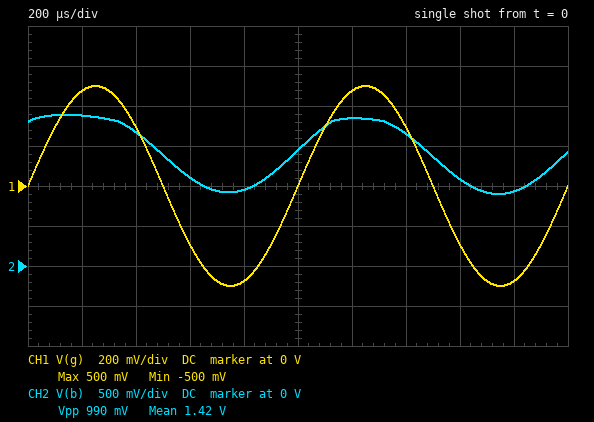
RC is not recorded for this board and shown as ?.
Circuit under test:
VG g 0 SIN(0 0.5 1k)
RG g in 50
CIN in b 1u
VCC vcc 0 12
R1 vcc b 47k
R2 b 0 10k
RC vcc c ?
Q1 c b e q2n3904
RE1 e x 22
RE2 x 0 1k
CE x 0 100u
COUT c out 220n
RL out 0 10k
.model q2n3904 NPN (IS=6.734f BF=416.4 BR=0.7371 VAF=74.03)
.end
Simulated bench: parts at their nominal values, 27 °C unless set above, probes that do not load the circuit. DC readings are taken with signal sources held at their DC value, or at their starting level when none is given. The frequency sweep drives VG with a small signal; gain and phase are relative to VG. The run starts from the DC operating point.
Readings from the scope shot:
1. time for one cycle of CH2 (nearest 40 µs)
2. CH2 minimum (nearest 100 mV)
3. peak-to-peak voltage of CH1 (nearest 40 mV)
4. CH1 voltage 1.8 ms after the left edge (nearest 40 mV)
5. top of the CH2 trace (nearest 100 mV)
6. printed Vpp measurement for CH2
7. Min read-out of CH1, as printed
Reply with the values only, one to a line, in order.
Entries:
1.00 ms
900 mV
1.00 V
-480 mV
1.9 V
990 mV
-500 mV
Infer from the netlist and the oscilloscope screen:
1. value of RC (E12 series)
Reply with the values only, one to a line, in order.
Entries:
10 kΩ
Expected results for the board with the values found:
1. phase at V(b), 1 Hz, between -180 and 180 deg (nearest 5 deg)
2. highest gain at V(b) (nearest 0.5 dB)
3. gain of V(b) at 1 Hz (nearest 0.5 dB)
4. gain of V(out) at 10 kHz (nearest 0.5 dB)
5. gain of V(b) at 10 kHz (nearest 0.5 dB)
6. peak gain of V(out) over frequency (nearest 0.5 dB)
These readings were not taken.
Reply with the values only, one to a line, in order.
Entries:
65 deg
-5.0 dB
-46.0 dB
15.5 dB
-5.0 dB
15.5 dB
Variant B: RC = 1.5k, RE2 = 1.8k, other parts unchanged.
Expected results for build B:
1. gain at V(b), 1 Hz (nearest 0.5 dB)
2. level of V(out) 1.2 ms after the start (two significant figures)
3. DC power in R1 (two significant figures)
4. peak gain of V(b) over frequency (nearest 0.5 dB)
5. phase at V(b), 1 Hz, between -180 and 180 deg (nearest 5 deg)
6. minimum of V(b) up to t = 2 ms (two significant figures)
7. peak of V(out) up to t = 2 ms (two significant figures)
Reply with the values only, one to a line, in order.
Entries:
-26.0 dB
-8.1 V
2.1 mW
0 dB
85 deg
1.4 V
2.3 V
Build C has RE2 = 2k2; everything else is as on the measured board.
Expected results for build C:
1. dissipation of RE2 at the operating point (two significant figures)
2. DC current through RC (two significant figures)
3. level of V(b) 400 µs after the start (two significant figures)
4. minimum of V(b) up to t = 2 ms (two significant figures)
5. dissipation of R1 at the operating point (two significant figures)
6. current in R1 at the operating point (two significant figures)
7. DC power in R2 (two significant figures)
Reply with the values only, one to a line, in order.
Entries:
920 µW
650 µA
2.0 V
1.2 V
2.1 mW
210 µA
440 µW
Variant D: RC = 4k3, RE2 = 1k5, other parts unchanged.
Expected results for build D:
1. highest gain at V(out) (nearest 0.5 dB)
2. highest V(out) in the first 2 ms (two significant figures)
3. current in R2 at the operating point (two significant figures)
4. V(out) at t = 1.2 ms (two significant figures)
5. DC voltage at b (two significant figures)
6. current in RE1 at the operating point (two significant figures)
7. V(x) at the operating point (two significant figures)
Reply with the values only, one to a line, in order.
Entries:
35.5 dB
3.4 V
210 µA
-6.3 V
2.1 V
940 µA
1.4 V
